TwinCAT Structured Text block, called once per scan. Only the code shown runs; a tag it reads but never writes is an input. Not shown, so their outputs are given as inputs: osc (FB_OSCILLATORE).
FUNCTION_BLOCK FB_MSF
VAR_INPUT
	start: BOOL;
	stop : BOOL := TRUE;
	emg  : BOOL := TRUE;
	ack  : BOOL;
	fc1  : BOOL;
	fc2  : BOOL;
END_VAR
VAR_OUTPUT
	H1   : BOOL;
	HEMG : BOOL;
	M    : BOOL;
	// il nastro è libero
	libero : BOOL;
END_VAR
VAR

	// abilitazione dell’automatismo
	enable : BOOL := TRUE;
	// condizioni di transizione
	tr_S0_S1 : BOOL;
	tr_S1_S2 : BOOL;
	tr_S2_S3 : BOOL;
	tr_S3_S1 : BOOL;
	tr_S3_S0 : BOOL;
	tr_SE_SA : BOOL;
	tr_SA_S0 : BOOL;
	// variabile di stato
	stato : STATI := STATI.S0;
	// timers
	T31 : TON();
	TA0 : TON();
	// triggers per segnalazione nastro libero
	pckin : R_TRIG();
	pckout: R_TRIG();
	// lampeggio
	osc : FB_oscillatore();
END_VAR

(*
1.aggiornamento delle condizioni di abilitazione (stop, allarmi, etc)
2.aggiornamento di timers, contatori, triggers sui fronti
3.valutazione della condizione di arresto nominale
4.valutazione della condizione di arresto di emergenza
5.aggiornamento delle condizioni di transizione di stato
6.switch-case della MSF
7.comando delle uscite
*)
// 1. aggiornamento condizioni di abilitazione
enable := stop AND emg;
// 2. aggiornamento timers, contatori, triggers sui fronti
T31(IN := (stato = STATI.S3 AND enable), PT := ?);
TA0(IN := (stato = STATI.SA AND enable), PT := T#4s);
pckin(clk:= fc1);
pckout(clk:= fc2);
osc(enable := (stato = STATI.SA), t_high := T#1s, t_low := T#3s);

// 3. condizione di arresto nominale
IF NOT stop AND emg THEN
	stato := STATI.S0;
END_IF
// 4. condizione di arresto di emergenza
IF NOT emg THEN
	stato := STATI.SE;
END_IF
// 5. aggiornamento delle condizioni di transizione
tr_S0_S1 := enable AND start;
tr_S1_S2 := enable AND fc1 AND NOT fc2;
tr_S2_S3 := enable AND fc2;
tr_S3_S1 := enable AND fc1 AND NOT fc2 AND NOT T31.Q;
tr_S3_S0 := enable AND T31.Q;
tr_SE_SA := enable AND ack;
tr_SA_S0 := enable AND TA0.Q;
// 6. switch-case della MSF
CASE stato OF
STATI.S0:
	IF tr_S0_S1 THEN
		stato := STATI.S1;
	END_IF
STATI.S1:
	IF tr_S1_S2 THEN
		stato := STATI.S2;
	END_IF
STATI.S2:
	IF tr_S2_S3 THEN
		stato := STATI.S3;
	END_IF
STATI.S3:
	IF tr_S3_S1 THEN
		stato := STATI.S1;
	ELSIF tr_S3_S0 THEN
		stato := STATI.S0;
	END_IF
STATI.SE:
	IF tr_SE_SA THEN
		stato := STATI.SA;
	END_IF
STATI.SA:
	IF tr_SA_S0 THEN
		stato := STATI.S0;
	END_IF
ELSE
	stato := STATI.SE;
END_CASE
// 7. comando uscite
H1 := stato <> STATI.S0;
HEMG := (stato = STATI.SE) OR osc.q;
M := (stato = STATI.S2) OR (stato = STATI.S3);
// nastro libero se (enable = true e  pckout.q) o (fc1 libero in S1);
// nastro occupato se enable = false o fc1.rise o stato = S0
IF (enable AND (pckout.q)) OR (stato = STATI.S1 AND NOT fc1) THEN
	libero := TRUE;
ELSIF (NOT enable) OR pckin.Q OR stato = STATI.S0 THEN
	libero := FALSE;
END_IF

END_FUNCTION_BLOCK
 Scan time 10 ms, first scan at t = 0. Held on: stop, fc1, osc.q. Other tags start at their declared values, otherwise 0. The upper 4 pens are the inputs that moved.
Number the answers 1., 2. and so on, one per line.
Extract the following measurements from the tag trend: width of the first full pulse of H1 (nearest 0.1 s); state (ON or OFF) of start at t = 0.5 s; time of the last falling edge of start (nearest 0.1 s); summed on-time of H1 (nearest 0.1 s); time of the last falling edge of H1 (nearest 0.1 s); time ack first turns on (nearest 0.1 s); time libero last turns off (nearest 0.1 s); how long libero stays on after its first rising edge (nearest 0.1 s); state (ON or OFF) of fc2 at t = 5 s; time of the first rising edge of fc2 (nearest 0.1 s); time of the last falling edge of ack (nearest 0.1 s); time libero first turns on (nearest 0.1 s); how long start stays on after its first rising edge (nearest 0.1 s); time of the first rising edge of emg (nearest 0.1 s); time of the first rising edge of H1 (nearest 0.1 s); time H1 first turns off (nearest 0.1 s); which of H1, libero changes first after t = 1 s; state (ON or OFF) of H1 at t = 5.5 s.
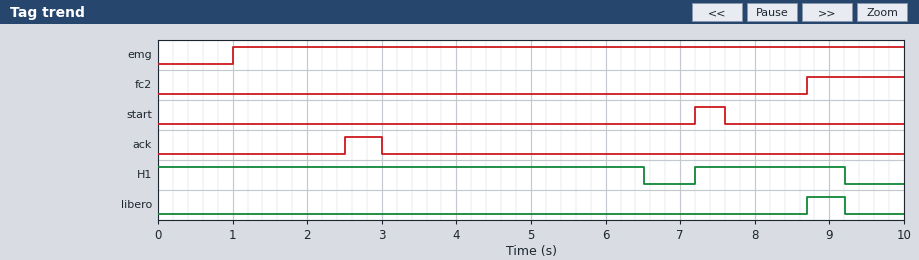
1. 2.0 s
2. OFF
3. 7.6 s
4. 8.5 s
5. 9.2 s
6. 2.5 s
7. 9.2 s
8. 0.5 s
9. OFF
10. 8.7 s
11. 3.0 s
12. 8.7 s
13. 0.4 s
14. 1.0 s
15. 7.2 s
16. 6.5 s
17. H1
18. ON
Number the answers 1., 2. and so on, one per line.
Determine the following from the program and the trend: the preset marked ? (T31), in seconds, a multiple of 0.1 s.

1. 0.5 s
